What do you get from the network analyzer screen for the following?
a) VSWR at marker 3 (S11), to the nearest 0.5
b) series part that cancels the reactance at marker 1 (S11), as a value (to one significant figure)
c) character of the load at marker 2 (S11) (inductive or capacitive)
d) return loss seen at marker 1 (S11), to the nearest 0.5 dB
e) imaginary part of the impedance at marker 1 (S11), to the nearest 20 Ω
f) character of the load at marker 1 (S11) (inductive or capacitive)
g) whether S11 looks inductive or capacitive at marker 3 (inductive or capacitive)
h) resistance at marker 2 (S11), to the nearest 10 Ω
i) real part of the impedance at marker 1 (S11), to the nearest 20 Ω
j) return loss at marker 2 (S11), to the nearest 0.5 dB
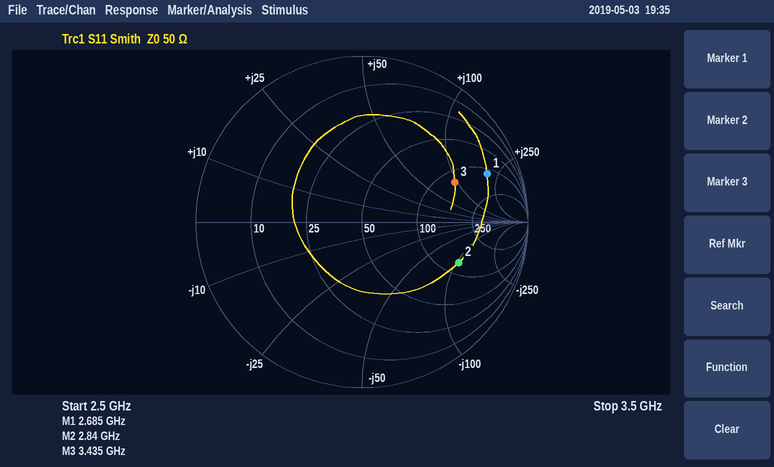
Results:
4.0
300 fF
capacitive
2.0 dB
+200 Ω
inductive
inductive
130 Ω
120 Ω
4.0 dB
